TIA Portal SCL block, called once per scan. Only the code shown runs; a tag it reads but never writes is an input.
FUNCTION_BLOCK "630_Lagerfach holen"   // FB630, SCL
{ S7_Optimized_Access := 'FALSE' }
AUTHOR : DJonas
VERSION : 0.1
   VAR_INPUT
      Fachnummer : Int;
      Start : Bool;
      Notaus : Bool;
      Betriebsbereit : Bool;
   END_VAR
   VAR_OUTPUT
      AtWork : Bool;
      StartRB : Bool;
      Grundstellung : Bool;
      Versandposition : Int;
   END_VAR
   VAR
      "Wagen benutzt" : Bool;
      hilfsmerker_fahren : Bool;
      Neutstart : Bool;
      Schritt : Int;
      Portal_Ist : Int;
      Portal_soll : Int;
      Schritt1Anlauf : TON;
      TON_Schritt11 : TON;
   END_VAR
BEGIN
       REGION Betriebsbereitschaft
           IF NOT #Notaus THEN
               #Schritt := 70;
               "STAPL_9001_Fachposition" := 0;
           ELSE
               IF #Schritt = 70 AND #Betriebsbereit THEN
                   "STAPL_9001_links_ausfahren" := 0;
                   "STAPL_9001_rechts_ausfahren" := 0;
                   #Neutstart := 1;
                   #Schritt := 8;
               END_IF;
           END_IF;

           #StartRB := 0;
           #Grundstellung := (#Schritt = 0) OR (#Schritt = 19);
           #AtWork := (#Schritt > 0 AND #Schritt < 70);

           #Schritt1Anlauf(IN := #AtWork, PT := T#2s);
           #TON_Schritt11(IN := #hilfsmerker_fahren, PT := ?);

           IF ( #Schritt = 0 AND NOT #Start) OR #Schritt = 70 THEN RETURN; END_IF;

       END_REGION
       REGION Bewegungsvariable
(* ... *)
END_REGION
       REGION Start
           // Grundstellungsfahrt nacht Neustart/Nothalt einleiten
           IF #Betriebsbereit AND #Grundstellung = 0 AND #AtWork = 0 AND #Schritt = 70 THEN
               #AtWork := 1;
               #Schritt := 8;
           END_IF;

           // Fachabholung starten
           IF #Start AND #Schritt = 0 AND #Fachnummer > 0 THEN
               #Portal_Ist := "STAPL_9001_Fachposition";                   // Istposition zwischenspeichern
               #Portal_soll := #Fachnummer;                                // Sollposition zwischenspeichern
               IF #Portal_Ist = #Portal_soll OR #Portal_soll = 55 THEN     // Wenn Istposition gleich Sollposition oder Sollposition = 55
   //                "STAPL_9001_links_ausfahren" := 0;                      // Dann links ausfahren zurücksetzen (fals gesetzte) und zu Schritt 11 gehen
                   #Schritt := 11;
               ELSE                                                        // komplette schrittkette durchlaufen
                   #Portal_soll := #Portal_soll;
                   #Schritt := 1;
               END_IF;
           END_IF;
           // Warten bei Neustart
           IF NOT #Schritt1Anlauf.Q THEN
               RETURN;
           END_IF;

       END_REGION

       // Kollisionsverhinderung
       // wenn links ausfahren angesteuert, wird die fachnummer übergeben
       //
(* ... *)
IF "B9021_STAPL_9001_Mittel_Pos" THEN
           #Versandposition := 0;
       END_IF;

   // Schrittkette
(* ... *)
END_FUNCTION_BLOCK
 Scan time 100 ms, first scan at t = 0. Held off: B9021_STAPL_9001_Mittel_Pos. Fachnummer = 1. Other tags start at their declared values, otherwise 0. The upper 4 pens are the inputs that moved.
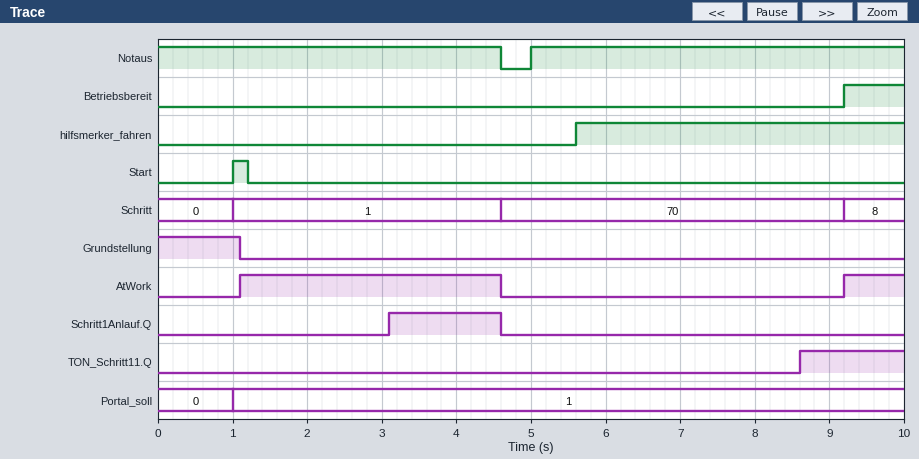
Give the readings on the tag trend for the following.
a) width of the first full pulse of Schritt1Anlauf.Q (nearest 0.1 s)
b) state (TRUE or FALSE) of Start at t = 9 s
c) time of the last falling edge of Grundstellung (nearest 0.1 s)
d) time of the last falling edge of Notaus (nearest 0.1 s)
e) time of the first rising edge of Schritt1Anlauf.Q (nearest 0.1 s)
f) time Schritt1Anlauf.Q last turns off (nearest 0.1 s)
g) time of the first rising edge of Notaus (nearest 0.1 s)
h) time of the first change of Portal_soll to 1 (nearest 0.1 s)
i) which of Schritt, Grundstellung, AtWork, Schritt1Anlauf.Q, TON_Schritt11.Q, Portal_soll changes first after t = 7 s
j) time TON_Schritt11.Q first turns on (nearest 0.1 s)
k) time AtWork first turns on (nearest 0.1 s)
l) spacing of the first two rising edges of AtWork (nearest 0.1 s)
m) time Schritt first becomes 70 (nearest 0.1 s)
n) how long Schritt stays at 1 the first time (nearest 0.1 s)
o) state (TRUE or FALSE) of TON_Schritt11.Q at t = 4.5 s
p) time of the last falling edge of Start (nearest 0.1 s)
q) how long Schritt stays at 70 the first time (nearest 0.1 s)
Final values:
1.5 s
FALSE
1.1 s
4.6 s
3.1 s
4.6 s
5.0 s
1.0 s
TON_Schritt11.Q
8.6 s
1.1 s
8.1 s
4.6 s
3.6 s
FALSE
1.2 s
4.6 s
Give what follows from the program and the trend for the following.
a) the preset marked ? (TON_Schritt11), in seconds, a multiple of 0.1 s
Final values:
3.0 s
